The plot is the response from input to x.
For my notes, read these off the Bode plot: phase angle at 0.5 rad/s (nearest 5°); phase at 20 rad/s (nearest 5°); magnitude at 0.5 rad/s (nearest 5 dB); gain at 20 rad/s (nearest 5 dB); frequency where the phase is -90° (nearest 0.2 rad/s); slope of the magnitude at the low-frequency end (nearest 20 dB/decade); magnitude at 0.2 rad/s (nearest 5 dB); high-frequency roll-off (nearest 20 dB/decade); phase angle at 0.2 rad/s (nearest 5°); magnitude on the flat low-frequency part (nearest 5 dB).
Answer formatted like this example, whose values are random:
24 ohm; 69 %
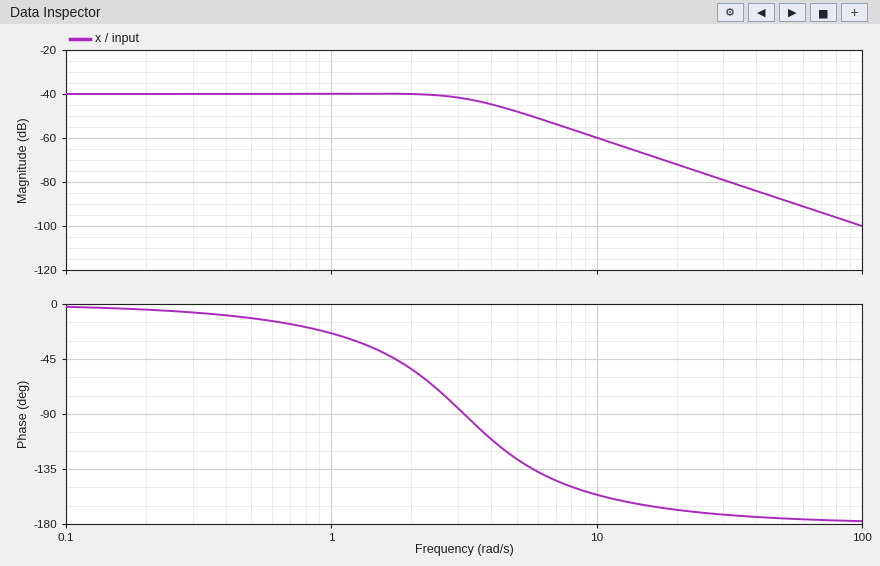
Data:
-10°; -170°; -40 dB; -70 dB; 3.2 rad/s; 0 dB/decade; -40 dB; -40 dB/decade; -5°; -40 dB
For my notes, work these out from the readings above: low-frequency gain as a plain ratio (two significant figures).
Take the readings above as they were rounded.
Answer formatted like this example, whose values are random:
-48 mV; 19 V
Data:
0.010
